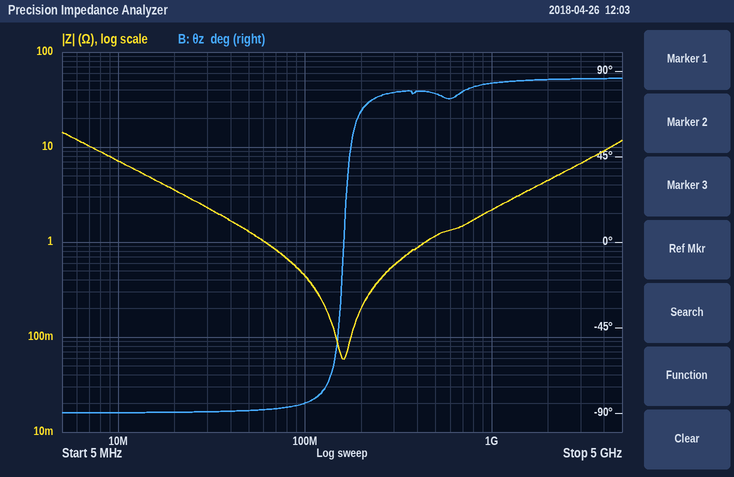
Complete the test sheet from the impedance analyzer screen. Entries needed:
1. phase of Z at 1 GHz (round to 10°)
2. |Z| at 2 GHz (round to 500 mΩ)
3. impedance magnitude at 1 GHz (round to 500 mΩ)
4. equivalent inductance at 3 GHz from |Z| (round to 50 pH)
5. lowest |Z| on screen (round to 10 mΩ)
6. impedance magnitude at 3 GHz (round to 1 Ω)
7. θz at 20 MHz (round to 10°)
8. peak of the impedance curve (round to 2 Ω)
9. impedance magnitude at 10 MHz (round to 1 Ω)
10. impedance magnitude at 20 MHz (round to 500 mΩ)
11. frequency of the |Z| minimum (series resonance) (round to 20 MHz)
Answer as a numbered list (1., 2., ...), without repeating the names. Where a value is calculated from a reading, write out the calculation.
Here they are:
1. 80°
2. 4.5 Ω
3. 2.0 Ω
4. L = 7 Ω/(2π × 3 GHz) ≈ 371 pH, so 350 pH to the nearest 50 pH
5. 60 mΩ
6. 7 Ω
7. -90°
8. 14 Ω
9. 7 Ω
10. 3.5 Ω
11. 160 MHz
